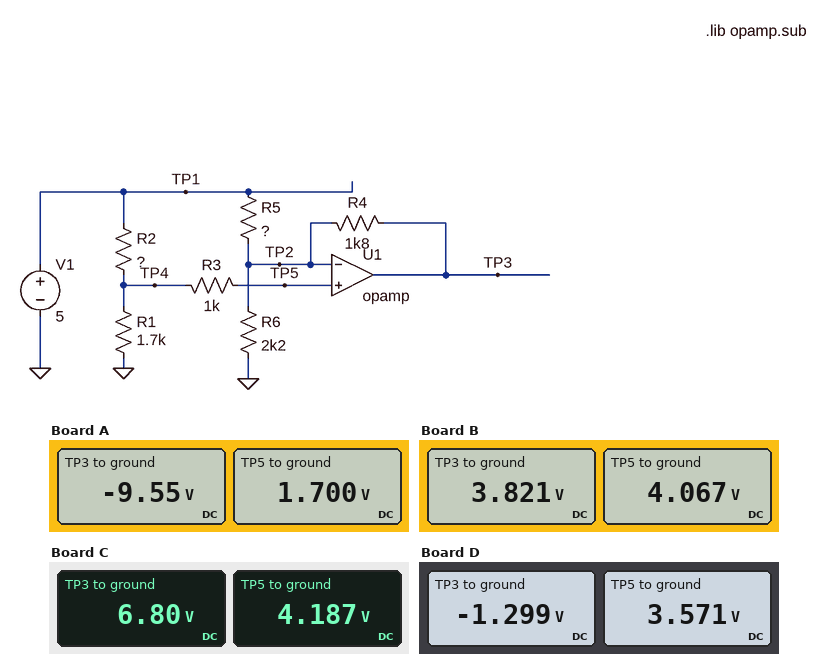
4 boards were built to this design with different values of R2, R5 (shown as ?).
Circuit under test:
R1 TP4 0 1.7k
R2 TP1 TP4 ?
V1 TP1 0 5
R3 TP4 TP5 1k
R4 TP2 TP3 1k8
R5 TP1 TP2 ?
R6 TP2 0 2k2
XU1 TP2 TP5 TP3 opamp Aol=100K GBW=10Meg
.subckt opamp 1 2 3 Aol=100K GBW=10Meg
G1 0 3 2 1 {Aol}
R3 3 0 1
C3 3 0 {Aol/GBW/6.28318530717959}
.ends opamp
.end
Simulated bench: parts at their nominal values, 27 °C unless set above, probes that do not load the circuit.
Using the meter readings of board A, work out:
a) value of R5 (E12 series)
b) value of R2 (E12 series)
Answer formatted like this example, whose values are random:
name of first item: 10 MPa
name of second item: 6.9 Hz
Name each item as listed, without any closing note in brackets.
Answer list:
value of R5: 470 Ω
value of R2: 3.3 kΩ
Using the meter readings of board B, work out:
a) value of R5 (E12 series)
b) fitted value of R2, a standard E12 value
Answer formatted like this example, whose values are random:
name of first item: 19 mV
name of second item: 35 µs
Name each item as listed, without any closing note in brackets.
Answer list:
value of R5: 470 Ω
fitted value of R2, a standard E12 value: 390 Ω
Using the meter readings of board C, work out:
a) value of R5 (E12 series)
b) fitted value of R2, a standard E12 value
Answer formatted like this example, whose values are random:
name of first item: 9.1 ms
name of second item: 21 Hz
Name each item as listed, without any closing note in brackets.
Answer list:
value of R5: 1.8 kΩ
fitted value of R2, a standard E12 value: 330 Ω
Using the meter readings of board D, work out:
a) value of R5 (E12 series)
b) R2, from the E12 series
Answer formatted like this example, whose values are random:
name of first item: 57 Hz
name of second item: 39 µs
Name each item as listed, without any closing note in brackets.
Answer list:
value of R5: 330 Ω
R2, from the E12 series: 680 Ω
